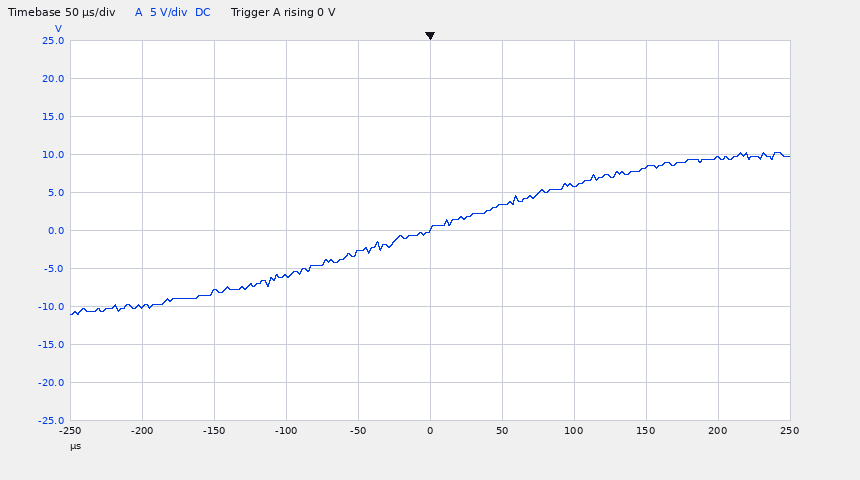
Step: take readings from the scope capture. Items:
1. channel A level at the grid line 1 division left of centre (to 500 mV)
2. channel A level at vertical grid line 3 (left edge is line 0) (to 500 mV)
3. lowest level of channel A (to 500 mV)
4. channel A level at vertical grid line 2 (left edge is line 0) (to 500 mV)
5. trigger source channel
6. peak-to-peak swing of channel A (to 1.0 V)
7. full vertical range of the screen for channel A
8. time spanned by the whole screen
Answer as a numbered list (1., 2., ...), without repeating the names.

1. -3.0 V
2. -6.0 V
3. -11.0 V
4. -8.0 V
5. channel A
6. 21.0 V
7. 50 V
8. 500 µs
